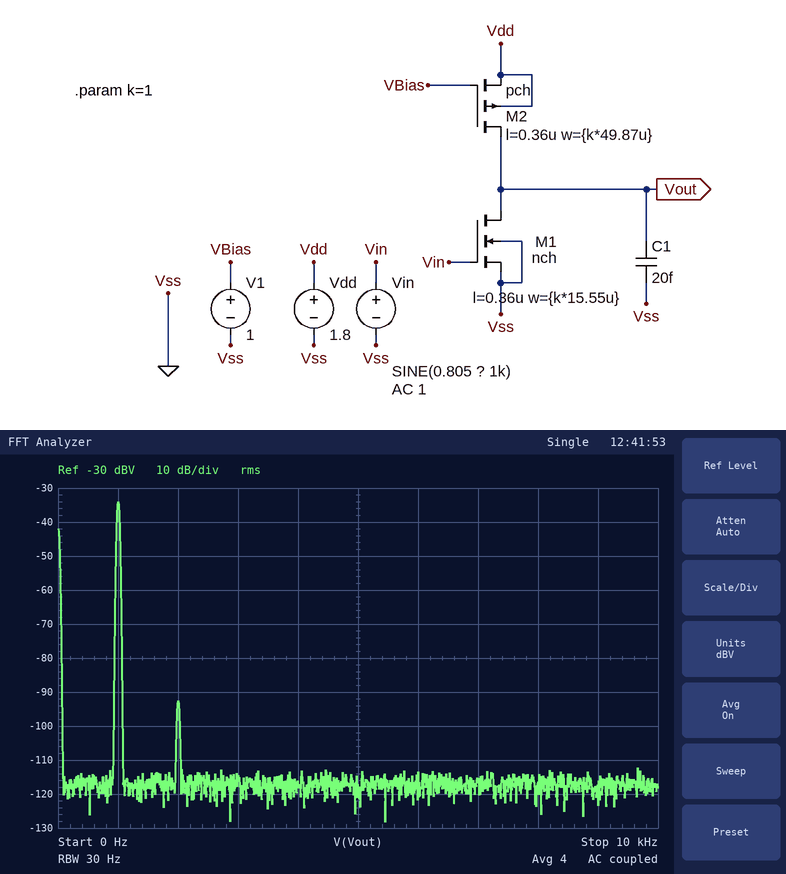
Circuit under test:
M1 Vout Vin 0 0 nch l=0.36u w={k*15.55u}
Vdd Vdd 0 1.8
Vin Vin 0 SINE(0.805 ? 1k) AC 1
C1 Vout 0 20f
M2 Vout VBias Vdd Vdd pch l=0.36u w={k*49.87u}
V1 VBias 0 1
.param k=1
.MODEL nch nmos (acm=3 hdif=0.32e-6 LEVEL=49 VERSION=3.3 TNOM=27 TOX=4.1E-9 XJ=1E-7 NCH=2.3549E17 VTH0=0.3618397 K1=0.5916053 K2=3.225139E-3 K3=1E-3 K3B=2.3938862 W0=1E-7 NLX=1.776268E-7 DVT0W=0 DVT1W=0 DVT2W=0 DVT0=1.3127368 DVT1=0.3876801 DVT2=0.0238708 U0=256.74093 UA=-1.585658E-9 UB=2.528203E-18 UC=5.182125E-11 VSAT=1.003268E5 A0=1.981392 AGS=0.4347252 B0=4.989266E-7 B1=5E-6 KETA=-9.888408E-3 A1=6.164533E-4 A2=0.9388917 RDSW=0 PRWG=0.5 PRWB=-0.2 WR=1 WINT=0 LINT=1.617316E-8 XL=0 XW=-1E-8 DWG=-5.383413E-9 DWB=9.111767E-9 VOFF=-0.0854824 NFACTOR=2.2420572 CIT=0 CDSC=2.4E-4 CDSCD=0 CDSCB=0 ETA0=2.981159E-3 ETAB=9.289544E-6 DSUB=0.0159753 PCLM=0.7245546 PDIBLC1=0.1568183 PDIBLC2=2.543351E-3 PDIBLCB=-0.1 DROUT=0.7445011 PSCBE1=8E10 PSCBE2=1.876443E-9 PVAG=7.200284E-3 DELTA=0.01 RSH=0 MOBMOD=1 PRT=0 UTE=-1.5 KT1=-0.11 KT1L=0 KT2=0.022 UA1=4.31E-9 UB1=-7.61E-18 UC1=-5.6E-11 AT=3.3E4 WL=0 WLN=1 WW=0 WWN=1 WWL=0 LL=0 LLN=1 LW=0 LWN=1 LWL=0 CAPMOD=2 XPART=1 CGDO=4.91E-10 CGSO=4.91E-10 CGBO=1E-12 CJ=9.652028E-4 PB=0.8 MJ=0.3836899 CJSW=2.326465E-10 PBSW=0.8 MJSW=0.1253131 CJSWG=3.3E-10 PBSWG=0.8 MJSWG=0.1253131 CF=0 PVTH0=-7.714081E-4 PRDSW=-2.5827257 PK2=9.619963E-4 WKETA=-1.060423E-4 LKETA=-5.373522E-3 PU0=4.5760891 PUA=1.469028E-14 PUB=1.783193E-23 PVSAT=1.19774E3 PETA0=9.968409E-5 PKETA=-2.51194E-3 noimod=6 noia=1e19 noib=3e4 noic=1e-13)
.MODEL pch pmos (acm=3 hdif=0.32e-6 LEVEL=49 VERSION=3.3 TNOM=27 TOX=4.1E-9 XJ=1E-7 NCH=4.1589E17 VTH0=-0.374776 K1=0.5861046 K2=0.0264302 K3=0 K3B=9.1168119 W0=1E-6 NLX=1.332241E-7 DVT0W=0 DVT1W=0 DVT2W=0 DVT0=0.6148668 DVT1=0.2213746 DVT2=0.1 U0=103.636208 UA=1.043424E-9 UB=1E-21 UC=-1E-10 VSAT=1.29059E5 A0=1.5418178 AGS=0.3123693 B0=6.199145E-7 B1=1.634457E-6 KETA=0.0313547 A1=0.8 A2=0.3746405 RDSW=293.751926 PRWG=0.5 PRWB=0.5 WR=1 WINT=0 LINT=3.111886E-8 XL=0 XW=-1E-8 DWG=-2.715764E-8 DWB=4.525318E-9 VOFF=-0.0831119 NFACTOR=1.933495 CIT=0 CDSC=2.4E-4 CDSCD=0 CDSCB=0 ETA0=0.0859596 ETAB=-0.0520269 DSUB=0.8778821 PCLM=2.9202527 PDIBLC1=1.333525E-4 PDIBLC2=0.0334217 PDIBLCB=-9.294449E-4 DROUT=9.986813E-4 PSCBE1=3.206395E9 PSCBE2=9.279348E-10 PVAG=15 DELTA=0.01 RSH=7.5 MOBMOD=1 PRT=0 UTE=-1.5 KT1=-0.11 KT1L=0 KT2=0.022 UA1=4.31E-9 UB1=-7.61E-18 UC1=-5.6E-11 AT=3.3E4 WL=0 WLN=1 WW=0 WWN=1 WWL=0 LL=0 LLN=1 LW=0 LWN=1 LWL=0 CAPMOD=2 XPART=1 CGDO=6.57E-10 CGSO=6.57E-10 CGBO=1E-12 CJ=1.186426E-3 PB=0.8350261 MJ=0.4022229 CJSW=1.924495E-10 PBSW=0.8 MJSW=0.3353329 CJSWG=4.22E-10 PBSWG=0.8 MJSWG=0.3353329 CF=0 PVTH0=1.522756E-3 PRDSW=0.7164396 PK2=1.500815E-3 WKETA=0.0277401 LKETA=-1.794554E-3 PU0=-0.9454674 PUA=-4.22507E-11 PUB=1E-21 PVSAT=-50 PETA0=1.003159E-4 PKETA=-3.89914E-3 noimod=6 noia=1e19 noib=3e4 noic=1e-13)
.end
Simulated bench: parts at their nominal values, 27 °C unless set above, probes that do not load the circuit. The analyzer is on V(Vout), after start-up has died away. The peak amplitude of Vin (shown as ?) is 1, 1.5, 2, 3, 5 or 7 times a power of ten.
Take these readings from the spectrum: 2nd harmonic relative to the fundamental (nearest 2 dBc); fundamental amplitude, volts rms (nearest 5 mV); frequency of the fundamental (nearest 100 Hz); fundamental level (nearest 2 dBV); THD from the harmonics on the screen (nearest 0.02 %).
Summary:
-58 dBc
20 mV
1.0 kHz
-34 dBV
0.12 %
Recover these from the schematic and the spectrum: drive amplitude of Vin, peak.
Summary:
1 mV
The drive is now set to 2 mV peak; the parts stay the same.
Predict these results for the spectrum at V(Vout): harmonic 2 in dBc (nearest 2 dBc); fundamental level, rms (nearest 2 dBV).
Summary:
-52 dBc
-28 dBV
